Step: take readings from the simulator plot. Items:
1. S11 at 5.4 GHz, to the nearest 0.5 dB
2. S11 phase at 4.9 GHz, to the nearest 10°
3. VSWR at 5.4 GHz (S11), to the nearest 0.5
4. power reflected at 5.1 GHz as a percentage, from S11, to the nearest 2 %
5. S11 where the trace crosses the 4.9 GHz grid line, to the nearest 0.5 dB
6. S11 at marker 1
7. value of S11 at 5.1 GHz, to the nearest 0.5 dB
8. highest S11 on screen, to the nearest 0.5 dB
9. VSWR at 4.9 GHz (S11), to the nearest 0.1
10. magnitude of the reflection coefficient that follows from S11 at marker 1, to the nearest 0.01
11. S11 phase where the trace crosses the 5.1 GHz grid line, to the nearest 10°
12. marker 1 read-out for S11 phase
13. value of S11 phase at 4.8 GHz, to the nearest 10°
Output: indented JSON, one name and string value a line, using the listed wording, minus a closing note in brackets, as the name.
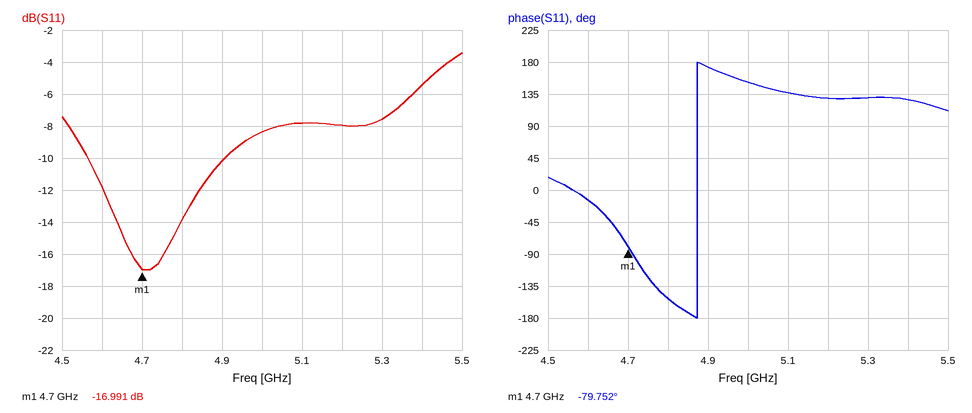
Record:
{
  "S11 at 5.4 GHz, to the nearest 0.5 dB": "-5.5 dB",
  "S11 phase at 4.9 GHz, to the nearest 10°": "170°",
  "VSWR at 5.4 GHz (S11), to the nearest 0.5": "3.5",
  "power reflected at 5.1 GHz as a percentage, from S11, to the nearest 2 %": "16 %",
  "S11 where the trace crosses the 4.9 GHz grid line, to the nearest 0.5 dB": "-10.0 dB",
  "S11 at marker 1": "-16.991 dB",
  "value of S11 at 5.1 GHz, to the nearest 0.5 dB": "-8.0 dB",
  "highest S11 on screen, to the nearest 0.5 dB": "-3.5 dB",
  "VSWR at 4.9 GHz (S11), to the nearest 0.1": "1.9",
  "magnitude of the reflection coefficient that follows from S11 at marker 1, to the nearest 0.01": "0.14",
  "S11 phase where the trace crosses the 5.1 GHz grid line, to the nearest 10°": "140°",
  "marker 1 read-out for S11 phase": "-79.752°",
  "value of S11 phase at 4.8 GHz, to the nearest 10°": "-150°"
}
